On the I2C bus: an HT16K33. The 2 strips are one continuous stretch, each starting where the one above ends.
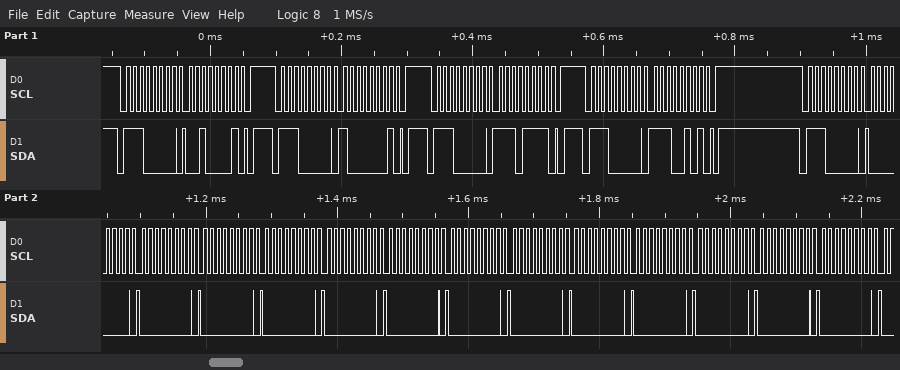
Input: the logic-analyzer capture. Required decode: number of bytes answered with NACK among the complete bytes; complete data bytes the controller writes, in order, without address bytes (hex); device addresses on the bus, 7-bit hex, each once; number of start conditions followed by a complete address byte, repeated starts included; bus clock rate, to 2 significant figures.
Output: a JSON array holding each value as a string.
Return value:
["0", "21 81 EF E5 00 00 00 00 00 00 00 00 00 00 00 00 00", "0x70", "5", "100 kHz"]
